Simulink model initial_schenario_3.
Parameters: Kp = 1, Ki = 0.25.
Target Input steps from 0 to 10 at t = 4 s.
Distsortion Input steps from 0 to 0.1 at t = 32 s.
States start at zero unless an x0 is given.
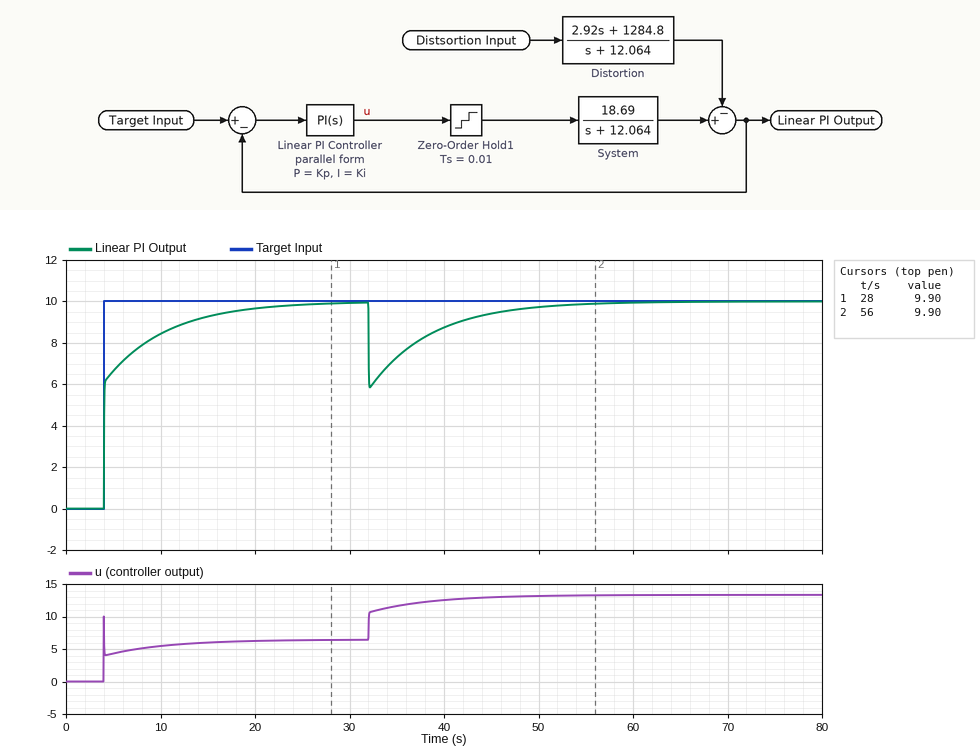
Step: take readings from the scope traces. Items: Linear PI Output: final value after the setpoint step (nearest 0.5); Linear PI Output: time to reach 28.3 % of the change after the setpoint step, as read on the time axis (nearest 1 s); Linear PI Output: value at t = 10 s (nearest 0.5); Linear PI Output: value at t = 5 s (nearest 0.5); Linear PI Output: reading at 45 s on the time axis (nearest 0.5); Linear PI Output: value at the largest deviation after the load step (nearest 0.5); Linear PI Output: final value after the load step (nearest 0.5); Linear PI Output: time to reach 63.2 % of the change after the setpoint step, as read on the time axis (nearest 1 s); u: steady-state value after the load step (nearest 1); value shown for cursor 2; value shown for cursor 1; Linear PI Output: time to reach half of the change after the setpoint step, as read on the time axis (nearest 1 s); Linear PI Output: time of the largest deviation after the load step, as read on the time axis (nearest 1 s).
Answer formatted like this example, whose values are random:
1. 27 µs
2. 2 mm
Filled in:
1. 10.0
2. 4 s
3. 8.5
4. 6.5
5. 9.5
6. 6.0
7. 10.0
8. 4 s
9. 13
10. 9.90
11. 9.90
12. 4 s
13. 32 s
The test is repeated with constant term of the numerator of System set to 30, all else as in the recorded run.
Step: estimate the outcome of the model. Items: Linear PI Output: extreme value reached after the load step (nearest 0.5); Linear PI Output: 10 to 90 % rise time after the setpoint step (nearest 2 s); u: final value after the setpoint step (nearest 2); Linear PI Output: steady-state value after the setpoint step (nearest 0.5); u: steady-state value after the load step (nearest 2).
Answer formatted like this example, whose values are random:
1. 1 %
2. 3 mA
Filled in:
1. 7.0
2. 6 s
3. 4
4. 10.0
5. 8
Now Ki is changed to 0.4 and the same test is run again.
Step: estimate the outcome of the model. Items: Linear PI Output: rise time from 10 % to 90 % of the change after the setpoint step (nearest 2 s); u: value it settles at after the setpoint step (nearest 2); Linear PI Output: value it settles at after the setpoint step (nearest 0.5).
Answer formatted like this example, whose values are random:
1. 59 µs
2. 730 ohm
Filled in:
1. 6 s
2. 6
3. 10.0
